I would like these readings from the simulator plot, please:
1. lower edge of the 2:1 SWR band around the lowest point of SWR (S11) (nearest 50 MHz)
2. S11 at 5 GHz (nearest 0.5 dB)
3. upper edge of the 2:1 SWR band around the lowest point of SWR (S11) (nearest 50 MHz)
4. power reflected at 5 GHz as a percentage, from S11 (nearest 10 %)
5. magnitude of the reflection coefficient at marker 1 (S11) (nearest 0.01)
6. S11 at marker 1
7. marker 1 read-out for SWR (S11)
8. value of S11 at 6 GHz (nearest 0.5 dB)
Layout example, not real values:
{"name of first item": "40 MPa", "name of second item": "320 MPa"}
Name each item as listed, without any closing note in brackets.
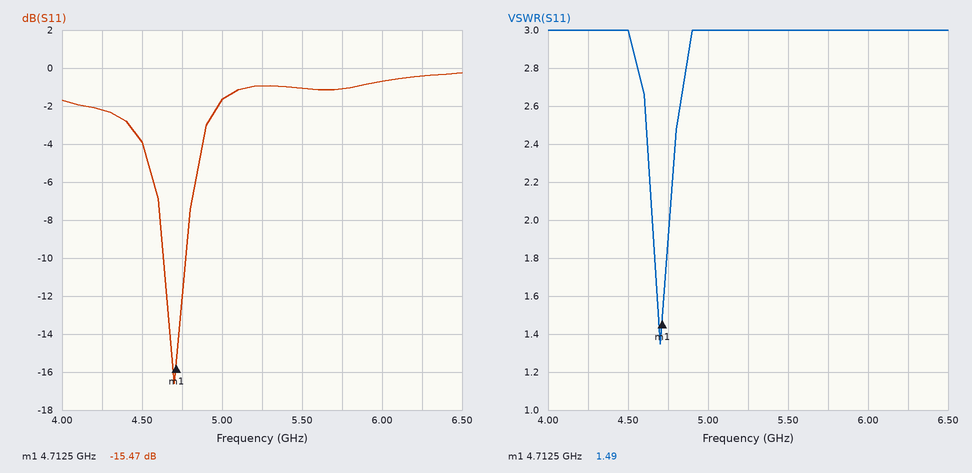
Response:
{"lower edge of the 2:1 SWR band around the lowest point of SWR (S11)": "4.65 GHz", "S11 at 5 GHz": "-1.5 dB", "upper edge of the 2:1 SWR band around the lowest point of SWR (S11)": "4.75 GHz", "power reflected at 5 GHz as a percentage, from S11": "70 %", "magnitude of the reflection coefficient at marker 1 (S11)": "0.17", "S11 at marker 1": "-15.47 dB", "marker 1 read-out for SWR": "1.49", "value of S11 at 6 GHz": "-0.5 dB"}
